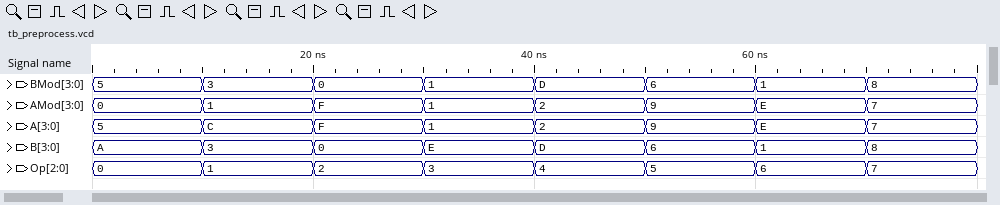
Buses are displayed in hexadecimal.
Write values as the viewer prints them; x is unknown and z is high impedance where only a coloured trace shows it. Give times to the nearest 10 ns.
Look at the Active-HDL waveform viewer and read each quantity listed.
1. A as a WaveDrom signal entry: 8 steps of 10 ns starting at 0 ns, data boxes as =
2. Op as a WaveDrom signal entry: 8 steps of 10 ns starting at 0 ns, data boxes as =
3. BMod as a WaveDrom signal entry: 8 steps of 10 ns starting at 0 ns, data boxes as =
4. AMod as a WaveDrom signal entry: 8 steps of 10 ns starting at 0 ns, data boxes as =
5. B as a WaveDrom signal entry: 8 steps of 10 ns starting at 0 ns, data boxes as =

{name: 'A', wave: '========', data: '5 C F 1 2 9 E 7'}
{name: 'Op', wave: '========', data: '0 1 2 3 4 5 6 7'}
{name: 'BMod', wave: '========', data: '5 3 0 1 D 6 1 8'}
{name: 'AMod', wave: '========', data: '0 1 F 1 2 9 E 7'}
{name: 'B', wave: '========', data: 'A 3 0 E D 6 1 8'}
